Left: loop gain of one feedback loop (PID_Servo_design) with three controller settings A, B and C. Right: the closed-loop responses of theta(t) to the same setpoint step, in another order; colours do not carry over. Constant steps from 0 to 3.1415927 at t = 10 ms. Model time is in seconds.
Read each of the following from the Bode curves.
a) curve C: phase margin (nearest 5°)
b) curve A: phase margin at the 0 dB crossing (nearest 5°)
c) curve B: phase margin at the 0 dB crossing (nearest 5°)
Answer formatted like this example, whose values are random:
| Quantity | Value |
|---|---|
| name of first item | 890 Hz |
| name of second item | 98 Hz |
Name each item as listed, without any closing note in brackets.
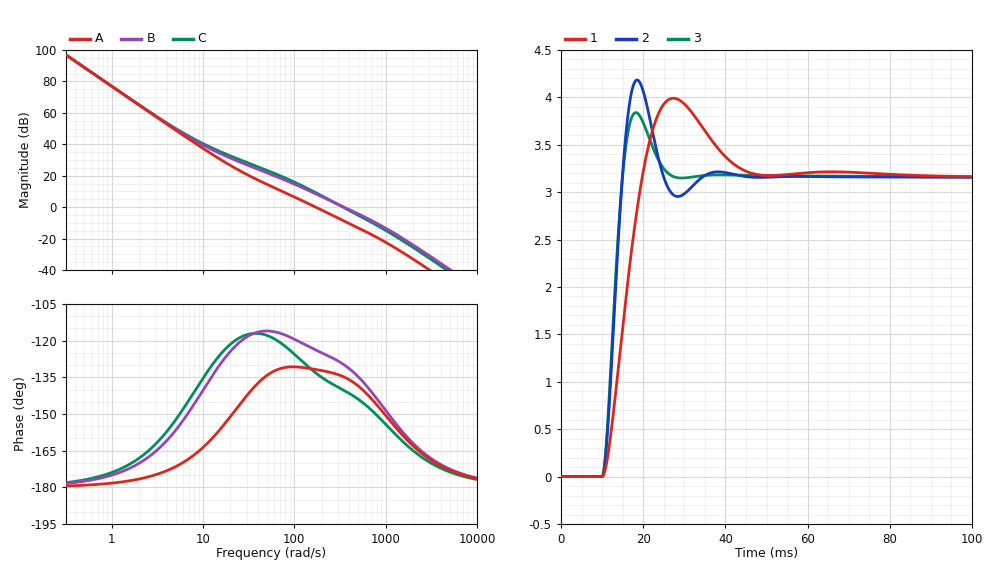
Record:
| Quantity | Value |
|---|---|
| curve C: phase margin | 40° |
| curve A: phase margin at the 0 dB crossing | 50° |
| curve B: phase margin at the 0 dB crossing | 50° |
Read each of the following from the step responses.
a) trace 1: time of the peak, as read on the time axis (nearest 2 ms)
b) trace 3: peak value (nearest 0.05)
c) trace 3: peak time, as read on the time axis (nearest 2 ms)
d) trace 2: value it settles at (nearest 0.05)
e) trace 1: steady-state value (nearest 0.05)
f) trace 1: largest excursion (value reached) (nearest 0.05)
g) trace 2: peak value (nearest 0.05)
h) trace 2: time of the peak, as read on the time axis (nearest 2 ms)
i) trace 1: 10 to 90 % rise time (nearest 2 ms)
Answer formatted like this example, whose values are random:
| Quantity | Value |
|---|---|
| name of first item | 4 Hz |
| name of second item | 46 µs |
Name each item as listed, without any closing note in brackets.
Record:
| Quantity | Value |
|---|---|
| trace 1: time of the peak, as read on the time axis | 28 ms |
| trace 3: peak value | 3.85 |
| trace 3: peak time, as read on the time axis | 18 ms |
| trace 2: value it settles at | 3.15 |
| trace 1: steady-state value | 3.15 |
| trace 1: largest excursion (value reached) | 4.00 |
| trace 2: peak value | 4.20 |
| trace 2: time of the peak, as read on the time axis | 18 ms |
| trace 1: 10 to 90 % rise time | 6 ms |
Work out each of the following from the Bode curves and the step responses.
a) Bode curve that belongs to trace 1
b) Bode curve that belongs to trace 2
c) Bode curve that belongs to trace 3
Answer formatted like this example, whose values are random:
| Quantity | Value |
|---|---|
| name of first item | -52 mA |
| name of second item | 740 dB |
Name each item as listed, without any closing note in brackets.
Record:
| Quantity | Value |
|---|---|
| Bode curve that belongs to trace 1 | A |
| Bode curve that belongs to trace 2 | C |
| Bode curve that belongs to trace 3 | B |
